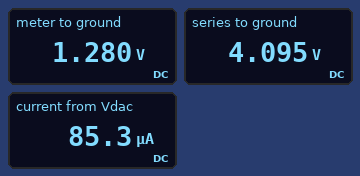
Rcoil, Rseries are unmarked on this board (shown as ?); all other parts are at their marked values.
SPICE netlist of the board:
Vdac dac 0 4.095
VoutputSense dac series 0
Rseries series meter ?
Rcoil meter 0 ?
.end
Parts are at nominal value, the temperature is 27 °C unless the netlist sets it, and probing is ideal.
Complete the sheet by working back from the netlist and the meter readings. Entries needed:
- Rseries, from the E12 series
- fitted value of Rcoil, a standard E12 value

33 kΩ
15 kΩ
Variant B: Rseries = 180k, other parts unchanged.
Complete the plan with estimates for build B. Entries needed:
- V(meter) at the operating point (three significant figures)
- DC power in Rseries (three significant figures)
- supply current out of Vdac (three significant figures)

315 mV
79.4 µW
21.0 µA
